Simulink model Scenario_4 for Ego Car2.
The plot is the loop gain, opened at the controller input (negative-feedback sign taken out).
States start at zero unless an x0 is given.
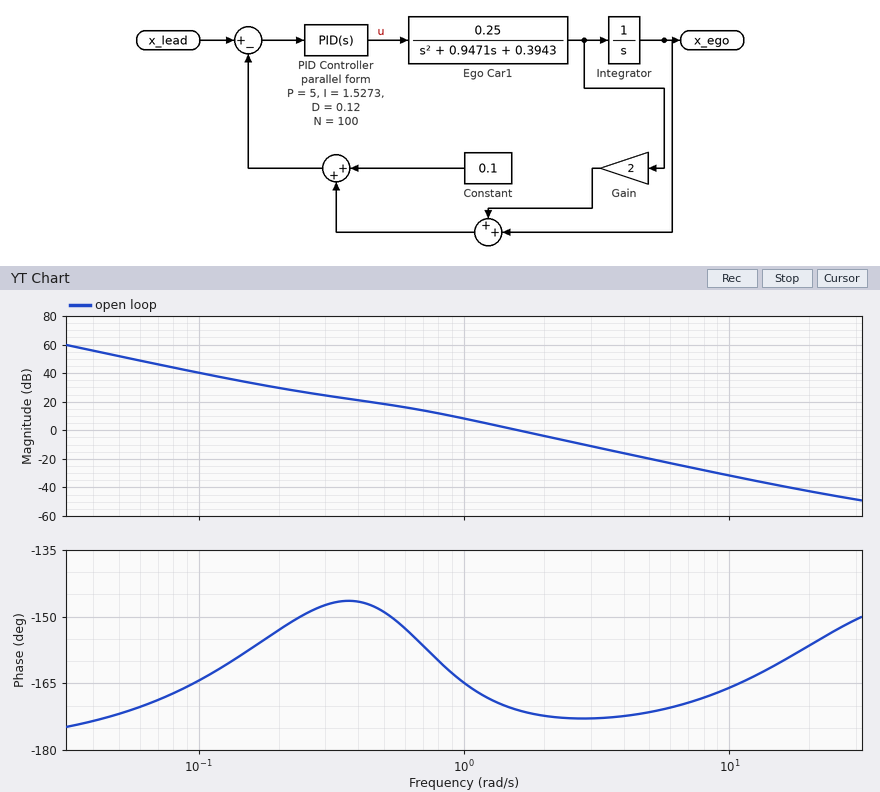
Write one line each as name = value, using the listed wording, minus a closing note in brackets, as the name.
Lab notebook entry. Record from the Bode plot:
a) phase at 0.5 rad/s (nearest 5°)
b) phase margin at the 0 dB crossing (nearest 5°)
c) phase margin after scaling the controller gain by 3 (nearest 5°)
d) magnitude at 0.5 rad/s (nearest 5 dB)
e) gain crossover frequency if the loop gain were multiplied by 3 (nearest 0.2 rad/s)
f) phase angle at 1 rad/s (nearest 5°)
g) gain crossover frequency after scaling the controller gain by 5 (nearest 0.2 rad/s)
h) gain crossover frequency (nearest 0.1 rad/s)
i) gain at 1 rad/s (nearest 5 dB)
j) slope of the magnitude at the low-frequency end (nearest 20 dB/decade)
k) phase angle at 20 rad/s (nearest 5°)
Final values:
phase at 0.5 rad/s = -150°
phase margin at the 0 dB crossing = 10°
phase margin after scaling the controller gain by 3 = 5°
magnitude at 0.5 rad/s = 20 dB
gain crossover frequency if the loop gain were multiplied by 3 = 2.8 rad/s
phase angle at 1 rad/s = -165°
gain crossover frequency after scaling the controller gain by 5 = 3.6 rad/s
gain crossover frequency = 1.6 rad/s
gain at 1 rad/s = 10 dB
slope of the magnitude at the low-frequency end = -40 dB/decade
phase angle at 20 rad/s = -155°
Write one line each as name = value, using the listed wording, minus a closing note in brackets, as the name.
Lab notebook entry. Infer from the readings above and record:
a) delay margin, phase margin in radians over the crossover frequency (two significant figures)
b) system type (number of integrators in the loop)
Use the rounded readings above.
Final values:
delay margin, phase margin in radians over the crossover frequency = 0.11 s
system type = 2
